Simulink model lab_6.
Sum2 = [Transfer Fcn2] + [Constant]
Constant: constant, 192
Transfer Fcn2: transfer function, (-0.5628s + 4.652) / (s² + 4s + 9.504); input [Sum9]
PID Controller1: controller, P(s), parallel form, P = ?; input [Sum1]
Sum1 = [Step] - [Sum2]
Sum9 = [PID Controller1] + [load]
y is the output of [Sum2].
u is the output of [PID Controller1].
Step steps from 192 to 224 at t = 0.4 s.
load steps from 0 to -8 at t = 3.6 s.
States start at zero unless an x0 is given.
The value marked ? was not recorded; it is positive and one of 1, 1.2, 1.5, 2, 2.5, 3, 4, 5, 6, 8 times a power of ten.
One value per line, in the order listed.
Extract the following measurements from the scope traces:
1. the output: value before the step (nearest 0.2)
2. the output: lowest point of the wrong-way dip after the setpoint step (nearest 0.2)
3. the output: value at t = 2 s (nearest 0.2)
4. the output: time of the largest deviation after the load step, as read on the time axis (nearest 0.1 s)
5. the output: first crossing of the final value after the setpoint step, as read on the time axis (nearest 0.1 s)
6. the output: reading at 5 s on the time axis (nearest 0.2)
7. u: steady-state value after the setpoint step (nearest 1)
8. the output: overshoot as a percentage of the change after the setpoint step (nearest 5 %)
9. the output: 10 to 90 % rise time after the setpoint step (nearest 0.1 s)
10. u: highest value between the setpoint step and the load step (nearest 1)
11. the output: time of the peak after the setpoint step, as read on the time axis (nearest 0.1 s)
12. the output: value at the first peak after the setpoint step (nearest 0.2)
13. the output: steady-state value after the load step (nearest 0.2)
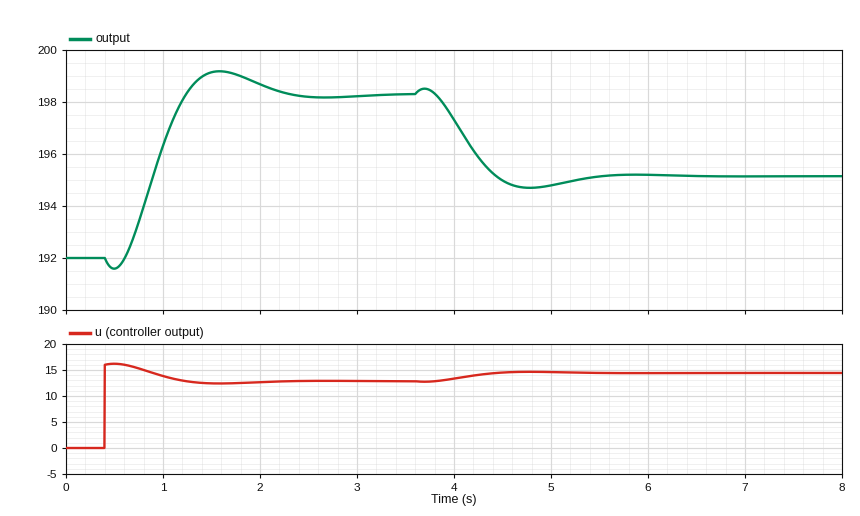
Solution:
192.0
191.6
198.6
4.8 s
1.2 s
194.8
13
15 %
0.5 s
16
1.6 s
199.2
195.2
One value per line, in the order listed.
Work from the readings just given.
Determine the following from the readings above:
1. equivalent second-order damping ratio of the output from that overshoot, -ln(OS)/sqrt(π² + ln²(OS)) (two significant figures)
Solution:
0.52
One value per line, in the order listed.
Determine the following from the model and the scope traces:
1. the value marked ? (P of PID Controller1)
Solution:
0.5
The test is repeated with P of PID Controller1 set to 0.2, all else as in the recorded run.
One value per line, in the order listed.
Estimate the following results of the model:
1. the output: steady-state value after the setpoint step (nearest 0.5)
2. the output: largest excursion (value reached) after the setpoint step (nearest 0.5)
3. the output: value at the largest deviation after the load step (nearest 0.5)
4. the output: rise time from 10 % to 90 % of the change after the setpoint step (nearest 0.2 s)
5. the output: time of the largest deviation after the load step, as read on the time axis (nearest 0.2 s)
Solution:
195.0
195.0
191.0
0.6 s
5.0 s
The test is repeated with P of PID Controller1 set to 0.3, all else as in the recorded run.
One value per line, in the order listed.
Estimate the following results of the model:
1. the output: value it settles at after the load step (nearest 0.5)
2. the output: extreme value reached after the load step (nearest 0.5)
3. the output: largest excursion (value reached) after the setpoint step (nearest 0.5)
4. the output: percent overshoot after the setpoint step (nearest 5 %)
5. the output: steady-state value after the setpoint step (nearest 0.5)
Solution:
192.5
192.5
196.5
10 %
196.0
